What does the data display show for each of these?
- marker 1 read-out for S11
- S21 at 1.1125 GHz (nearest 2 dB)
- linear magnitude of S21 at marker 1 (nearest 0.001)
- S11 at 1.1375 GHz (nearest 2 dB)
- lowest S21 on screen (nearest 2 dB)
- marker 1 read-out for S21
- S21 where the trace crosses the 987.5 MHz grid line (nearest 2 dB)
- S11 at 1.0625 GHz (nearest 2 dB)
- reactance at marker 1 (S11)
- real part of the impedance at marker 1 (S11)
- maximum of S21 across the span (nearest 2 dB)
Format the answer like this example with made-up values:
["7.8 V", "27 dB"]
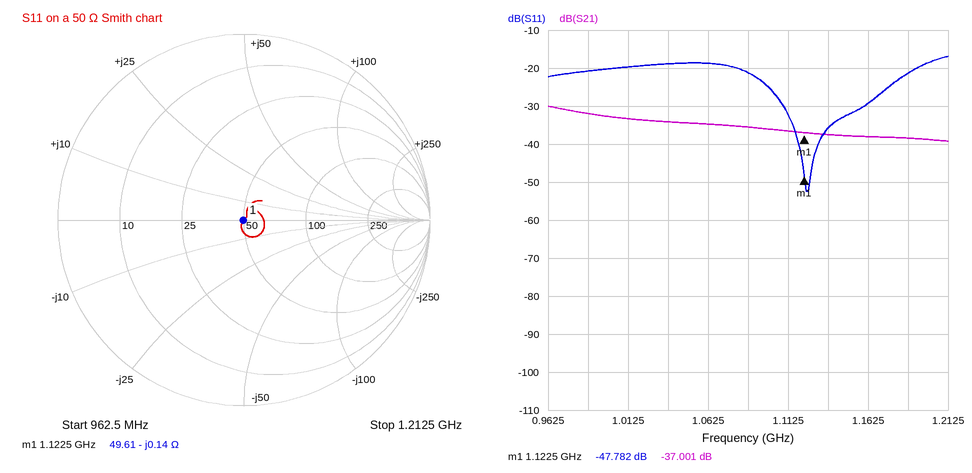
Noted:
["-47.782 dB", "-36 dB", "0.014", "-36 dB", "-40 dB", "-37.001 dB", "-32 dB", "-18 dB", "-0.14 Ω", "49.61 Ω", "-30 dB"]
